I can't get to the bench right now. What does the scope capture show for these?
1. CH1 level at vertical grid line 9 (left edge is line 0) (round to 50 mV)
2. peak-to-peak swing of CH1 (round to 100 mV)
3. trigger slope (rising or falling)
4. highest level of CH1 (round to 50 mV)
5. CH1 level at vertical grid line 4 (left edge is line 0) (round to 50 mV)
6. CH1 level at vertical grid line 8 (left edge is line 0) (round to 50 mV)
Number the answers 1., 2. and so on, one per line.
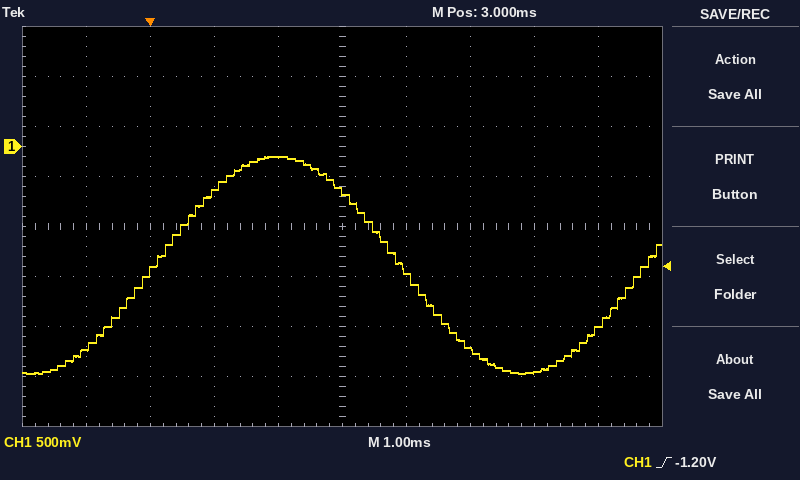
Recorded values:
1. -1.80 V
2. 2.20 V
3. rising
4. -100 mV
5. -100 mV
6. -2.25 V
